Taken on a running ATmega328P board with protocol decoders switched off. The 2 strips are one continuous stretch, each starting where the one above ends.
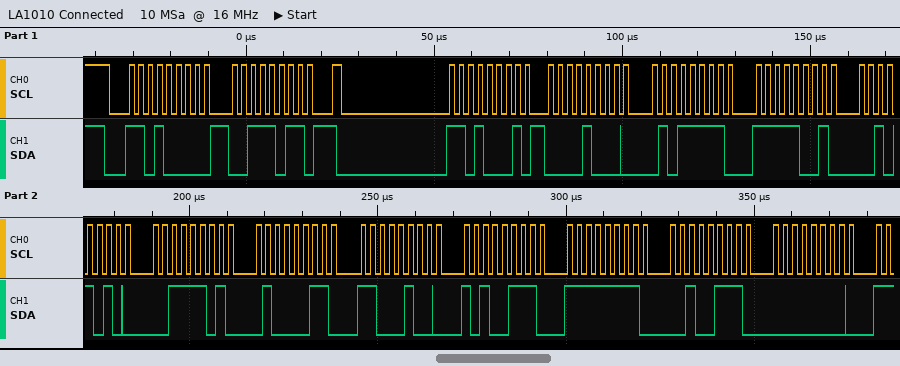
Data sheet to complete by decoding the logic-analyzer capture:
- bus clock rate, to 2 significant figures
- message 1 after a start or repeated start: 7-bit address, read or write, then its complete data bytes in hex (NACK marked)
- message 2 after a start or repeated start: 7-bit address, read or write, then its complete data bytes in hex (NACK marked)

400 kHz
0x68 write: 3B
0x68 read: 08 5F F9 2A 3D 43 C4 A7 FF 27 00
